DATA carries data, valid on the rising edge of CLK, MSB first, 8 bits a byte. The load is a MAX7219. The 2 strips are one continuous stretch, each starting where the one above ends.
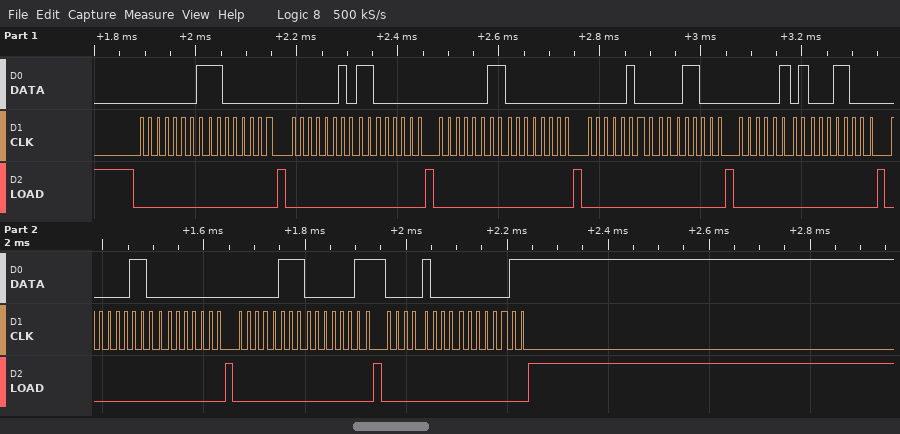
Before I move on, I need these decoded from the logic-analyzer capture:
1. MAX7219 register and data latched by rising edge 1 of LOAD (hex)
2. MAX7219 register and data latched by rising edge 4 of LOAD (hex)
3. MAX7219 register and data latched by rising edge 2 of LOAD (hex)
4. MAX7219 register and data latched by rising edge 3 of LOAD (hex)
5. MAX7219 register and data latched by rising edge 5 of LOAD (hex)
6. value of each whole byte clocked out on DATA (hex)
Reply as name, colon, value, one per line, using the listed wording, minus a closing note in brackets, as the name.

MAX7219 register and data latched by rising edge 1 of LOAD: register 0x1, data 0xC0
MAX7219 register and data latched by rising edge 4 of LOAD: register 0x4, data 0x18
MAX7219 register and data latched by rising edge 2 of LOAD: register 0x2, data 0xC0
MAX7219 register and data latched by rising edge 3 of LOAD: register 0x3, data 0x00
MAX7219 register and data latched by rising edge 5 of LOAD: register 0x5, data 0x18
value of each whole byte clocked out on DATA: 01 C0 02 C0 03 00 04 18 05 18 06 00 07 03 08 03
